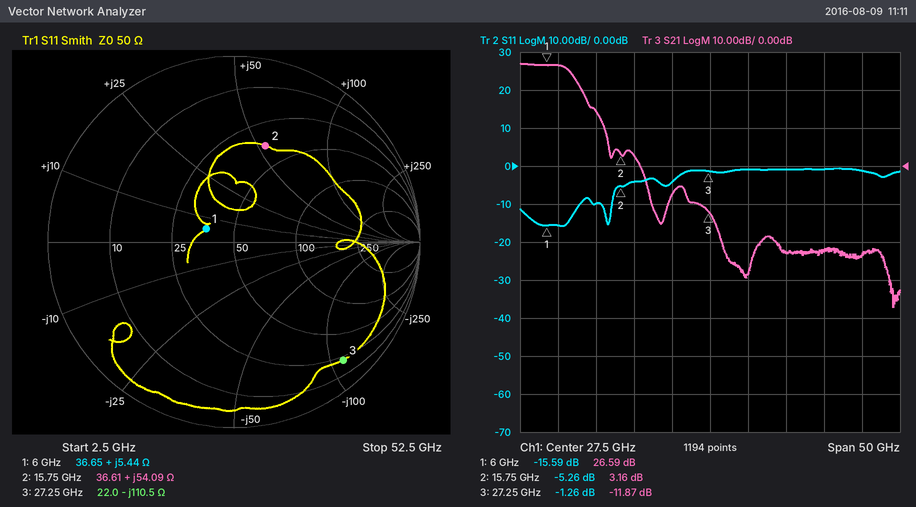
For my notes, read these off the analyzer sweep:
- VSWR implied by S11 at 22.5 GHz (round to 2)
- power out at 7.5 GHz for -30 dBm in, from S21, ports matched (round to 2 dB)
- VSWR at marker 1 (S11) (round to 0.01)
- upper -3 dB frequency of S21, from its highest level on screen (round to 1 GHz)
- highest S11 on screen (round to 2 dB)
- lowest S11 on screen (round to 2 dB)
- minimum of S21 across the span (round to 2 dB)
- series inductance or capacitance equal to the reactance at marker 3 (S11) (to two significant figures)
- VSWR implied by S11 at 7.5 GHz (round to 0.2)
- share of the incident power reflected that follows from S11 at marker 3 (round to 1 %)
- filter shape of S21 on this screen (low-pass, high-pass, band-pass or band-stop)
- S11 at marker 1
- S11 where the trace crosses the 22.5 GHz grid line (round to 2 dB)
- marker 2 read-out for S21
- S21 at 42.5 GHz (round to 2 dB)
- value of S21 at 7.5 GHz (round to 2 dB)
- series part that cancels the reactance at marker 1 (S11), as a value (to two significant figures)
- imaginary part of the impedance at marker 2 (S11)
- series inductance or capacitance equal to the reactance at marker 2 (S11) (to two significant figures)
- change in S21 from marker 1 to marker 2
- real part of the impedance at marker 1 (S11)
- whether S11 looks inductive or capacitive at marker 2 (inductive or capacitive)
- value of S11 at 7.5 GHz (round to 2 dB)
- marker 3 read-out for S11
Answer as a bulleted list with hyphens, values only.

- 4
- -4 dBm
- 1.40
- 9 GHz
- 0 dB
- -16 dB
- -38 dB
- 53 fF
- 1.4
- 75 %
- low-pass
- -15.59 dB
- -4 dB
- 3.16 dB
- -22 dB
- 26 dB
- 4.9 pF
- +54.09 Ω
- 550 pH
- -23.43 dB
- 36.65 Ω
- inductive
- -16 dB
- -1.26 dB
